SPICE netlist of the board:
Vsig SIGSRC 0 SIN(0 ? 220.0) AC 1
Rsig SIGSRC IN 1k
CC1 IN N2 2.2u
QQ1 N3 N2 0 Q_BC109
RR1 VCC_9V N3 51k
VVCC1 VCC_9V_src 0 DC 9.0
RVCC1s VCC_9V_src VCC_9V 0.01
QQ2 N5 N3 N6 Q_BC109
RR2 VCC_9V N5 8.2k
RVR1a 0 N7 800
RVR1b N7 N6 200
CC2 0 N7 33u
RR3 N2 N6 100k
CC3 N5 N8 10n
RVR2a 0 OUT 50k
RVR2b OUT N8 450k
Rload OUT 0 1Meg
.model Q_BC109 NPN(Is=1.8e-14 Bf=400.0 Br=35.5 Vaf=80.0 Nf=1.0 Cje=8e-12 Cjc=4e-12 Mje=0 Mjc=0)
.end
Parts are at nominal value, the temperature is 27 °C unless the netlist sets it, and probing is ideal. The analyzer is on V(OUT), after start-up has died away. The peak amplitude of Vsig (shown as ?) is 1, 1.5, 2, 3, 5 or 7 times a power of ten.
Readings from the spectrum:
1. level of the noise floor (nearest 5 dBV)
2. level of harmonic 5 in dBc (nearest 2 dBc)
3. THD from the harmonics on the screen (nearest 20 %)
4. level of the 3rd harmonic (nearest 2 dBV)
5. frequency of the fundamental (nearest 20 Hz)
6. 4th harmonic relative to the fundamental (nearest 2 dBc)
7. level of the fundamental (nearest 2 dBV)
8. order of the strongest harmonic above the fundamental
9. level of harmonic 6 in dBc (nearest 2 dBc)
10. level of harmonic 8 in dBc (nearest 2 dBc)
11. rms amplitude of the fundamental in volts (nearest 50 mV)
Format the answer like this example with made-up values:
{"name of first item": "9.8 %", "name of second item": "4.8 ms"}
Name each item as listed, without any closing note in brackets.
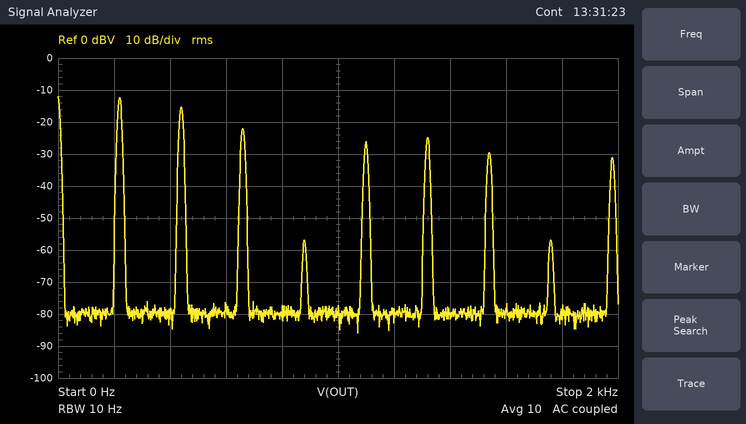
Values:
{"level of the noise floor": "-80 dBV", "level of harmonic 5 in dBc": "-14 dBc", "THD from the harmonics on the screen": "80 %", "level of the 3rd harmonic": "-22 dBV", "frequency of the fundamental": "220 Hz", "4th harmonic relative to the fundamental": "-44 dBc", "level of the fundamental": "-12 dBV", "order of the strongest harmonic above the fundamental": "2", "level of harmonic 6 in dBc": "-12 dBc", "level of harmonic 8 in dBc": "-44 dBc", "rms amplitude of the fundamental in volts": "250 mV"}
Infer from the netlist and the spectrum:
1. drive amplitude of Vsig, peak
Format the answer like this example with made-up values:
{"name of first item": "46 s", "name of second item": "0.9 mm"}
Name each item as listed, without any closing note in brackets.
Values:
{"drive amplitude of Vsig, peak": "300 mV"}
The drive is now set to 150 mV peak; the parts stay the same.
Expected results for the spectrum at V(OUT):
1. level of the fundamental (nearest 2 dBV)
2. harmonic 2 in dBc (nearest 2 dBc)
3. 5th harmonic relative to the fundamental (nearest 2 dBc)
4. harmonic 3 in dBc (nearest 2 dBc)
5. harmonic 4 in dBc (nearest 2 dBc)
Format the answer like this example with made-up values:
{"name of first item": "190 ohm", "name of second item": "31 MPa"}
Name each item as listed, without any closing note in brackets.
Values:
{"level of the fundamental": "-12 dBV", "harmonic 2 in dBc": "-4 dBc", "5th harmonic relative to the fundamental": "-12 dBc", "harmonic 3 in dBc": "-16 dBc", "harmonic 4 in dBc": "-16 dBc"}
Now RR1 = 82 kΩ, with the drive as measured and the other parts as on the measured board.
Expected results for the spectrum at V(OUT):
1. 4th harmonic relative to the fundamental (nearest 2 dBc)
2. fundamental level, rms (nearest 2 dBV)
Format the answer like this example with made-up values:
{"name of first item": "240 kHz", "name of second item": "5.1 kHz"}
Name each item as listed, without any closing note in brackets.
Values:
{"4th harmonic relative to the fundamental": "-26 dBc", "fundamental level, rms": "-12 dBV"}
